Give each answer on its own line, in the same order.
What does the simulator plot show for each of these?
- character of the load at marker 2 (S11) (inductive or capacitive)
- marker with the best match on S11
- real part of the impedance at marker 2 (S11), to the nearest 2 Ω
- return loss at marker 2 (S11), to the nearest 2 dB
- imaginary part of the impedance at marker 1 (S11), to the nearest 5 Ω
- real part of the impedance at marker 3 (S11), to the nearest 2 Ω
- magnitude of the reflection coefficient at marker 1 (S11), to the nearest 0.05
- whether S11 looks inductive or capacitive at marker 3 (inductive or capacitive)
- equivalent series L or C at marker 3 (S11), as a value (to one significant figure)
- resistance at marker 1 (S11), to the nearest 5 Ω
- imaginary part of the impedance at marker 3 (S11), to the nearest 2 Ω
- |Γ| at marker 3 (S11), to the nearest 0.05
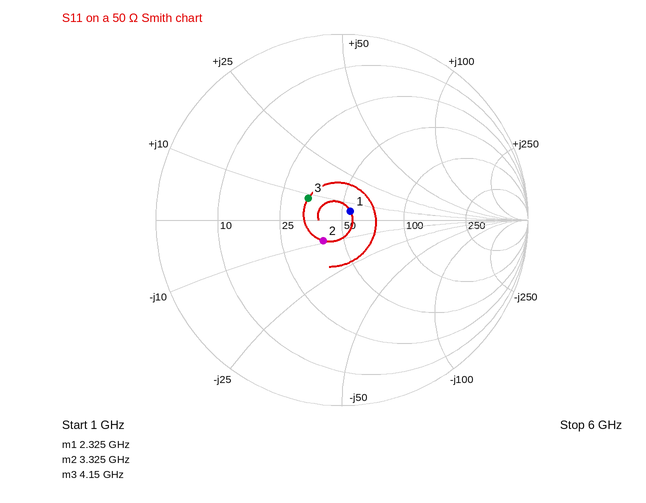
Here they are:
capacitive
marker 1
40 Ω
16 dB
+5 Ω
34 Ω
0.05
inductive
300 pH
55 Ω
+8 Ω
0.20
